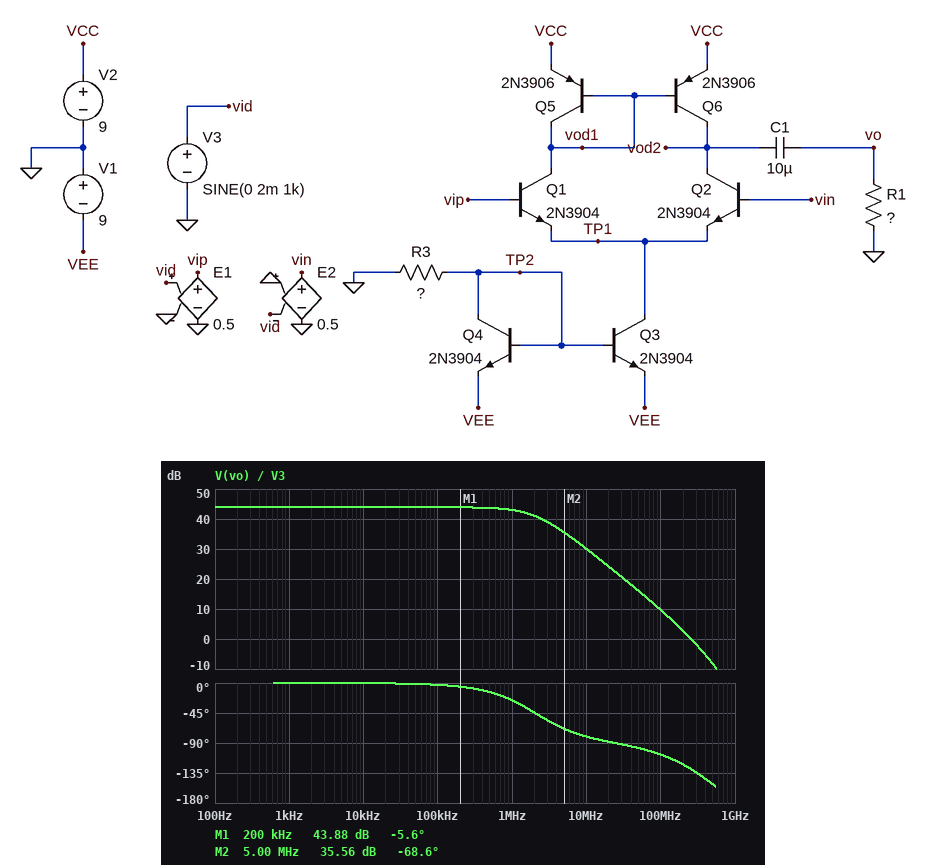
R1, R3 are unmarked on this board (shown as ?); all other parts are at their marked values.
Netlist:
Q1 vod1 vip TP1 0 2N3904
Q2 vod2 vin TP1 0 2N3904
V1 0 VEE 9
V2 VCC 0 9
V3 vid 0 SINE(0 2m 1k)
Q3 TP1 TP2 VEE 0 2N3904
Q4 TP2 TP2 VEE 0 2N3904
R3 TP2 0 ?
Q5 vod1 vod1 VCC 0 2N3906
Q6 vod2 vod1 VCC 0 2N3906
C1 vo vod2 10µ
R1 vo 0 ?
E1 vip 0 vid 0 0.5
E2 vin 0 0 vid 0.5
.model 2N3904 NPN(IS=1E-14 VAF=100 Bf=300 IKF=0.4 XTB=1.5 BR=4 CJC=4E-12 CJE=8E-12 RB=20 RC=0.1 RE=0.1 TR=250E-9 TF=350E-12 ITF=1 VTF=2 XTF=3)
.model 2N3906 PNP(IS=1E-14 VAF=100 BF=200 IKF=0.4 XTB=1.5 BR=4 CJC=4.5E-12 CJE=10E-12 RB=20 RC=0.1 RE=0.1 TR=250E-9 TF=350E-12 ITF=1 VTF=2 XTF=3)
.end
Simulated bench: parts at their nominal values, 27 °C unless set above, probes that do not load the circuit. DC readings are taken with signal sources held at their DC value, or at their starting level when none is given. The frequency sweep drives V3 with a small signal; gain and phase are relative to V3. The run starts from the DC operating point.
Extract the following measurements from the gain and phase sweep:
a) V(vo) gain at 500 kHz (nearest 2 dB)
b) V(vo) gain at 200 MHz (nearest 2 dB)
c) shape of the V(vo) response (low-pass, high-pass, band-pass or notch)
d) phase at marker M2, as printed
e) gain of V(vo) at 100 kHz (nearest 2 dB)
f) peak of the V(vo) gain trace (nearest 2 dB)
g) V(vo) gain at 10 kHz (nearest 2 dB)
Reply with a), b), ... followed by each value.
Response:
a) 44 dB
b) 2 dB
c) low-pass
d) -68.6 deg
e) 44 dB
f) 44 dB
g) 44 dB
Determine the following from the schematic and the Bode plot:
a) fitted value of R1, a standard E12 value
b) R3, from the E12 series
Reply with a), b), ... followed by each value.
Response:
a) 6.8 kΩ
b) 6.8 kΩ
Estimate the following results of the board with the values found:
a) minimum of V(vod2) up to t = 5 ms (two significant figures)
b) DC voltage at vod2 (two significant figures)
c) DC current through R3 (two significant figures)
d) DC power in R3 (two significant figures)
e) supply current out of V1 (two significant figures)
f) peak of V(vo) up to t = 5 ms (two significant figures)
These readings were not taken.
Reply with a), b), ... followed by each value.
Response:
a) 7.5 V
b) 7.8 V
c) 1.2 mA
d) 10 mW
e) 2.5 mA
f) 310 mV
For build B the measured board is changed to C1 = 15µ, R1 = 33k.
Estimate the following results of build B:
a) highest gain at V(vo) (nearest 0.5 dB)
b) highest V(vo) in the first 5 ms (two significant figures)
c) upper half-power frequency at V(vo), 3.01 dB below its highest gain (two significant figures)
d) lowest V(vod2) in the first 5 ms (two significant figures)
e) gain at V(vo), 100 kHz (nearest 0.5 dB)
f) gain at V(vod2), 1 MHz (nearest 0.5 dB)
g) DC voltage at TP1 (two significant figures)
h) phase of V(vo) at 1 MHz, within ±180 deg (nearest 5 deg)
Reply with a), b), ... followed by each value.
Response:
a) 55.5 dB
b) 1.0 V
c) 560 kHz
d) 6.7 V
e) 55.0 dB
f) 49.0 dB
g) -640 mV
h) -60 deg
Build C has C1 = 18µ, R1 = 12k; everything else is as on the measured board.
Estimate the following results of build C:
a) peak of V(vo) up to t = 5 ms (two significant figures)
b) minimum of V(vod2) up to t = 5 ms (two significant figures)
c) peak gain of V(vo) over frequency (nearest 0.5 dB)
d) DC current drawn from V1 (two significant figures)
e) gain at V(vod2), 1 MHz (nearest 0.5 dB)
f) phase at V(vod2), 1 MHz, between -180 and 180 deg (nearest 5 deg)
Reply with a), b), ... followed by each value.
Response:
a) 520 mV
b) 7.3 V
c) 48.5 dB
d) 2.5 mA
e) 46.0 dB
f) -40 deg
